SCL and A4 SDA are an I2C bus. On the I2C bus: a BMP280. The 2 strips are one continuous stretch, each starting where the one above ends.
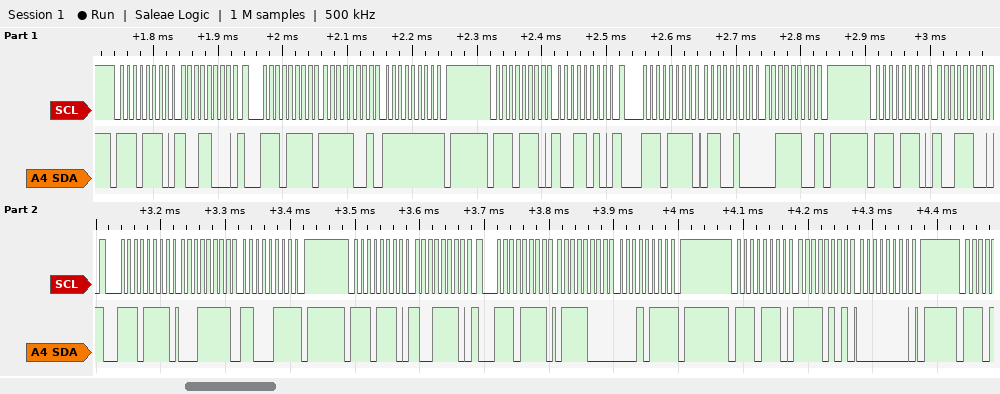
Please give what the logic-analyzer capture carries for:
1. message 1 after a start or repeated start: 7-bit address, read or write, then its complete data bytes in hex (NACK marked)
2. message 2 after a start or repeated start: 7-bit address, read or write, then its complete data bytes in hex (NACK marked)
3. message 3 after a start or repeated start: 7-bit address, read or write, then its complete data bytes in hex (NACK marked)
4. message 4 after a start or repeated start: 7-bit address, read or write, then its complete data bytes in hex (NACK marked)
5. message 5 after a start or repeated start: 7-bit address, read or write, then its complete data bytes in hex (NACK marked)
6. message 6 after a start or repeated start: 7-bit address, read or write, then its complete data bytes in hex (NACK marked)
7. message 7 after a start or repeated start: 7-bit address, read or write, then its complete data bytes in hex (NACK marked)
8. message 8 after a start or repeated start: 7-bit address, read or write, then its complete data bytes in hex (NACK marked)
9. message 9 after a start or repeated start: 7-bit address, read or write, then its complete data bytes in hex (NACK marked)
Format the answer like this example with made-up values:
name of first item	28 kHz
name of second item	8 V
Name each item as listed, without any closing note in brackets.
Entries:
message 1 after a start or repeated start: 7-bit address, read or write, then its complete data bytes in hex	0x77 write: 98
message 2 after a start or repeated start: 7-bit address, read or write, then its complete data bytes in hex	0x77 read: F9 FF NACK
message 3 after a start or repeated start: 7-bit address, read or write, then its complete data bytes in hex	0x77 write: 9A
message 4 after a start or repeated start: 7-bit address, read or write, then its complete data bytes in hex	0x77 read: 64 3C NACK
message 5 after a start or repeated start: 7-bit address, read or write, then its complete data bytes in hex	0x77 write: 9C
message 6 after a start or repeated start: 7-bit address, read or write, then its complete data bytes in hex	0x77 read: 1F C7 NACK
message 7 after a start or repeated start: 7-bit address, read or write, then its complete data bytes in hex	0x77 write: 9E
message 8 after a start or repeated start: 7-bit address, read or write, then its complete data bytes in hex	0x77 read: 78 17 NACK
message 9 after a start or repeated start: 7-bit address, read or write, then its complete data bytes in hex	0x77 write: F5 00
